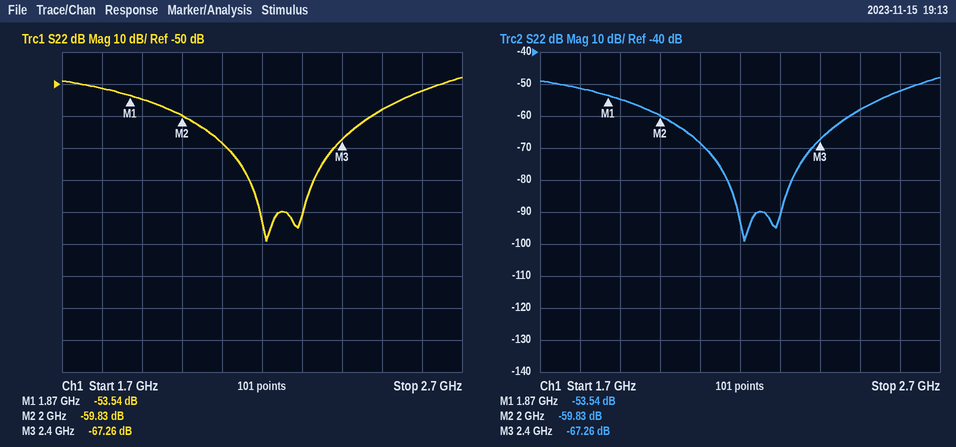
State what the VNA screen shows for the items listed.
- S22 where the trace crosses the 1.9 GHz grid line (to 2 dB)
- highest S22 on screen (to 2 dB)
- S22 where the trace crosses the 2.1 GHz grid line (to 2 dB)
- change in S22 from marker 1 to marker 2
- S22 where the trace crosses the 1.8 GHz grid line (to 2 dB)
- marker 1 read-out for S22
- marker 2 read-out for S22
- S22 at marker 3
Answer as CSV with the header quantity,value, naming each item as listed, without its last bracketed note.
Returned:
quantity,value
S22 where the trace crosses the 1.9 GHz grid line,-54 dB
highest S22 on screen,-48 dB
S22 where the trace crosses the 2.1 GHz grid line,-68 dB
change in S22 from marker 1 to marker 2,-6.29 dB
S22 where the trace crosses the 1.8 GHz grid line,-52 dB
marker 1 read-out for S22,-53.54 dB
marker 2 read-out for S22,-59.83 dB
S22 at marker 3,-67.26 dB
